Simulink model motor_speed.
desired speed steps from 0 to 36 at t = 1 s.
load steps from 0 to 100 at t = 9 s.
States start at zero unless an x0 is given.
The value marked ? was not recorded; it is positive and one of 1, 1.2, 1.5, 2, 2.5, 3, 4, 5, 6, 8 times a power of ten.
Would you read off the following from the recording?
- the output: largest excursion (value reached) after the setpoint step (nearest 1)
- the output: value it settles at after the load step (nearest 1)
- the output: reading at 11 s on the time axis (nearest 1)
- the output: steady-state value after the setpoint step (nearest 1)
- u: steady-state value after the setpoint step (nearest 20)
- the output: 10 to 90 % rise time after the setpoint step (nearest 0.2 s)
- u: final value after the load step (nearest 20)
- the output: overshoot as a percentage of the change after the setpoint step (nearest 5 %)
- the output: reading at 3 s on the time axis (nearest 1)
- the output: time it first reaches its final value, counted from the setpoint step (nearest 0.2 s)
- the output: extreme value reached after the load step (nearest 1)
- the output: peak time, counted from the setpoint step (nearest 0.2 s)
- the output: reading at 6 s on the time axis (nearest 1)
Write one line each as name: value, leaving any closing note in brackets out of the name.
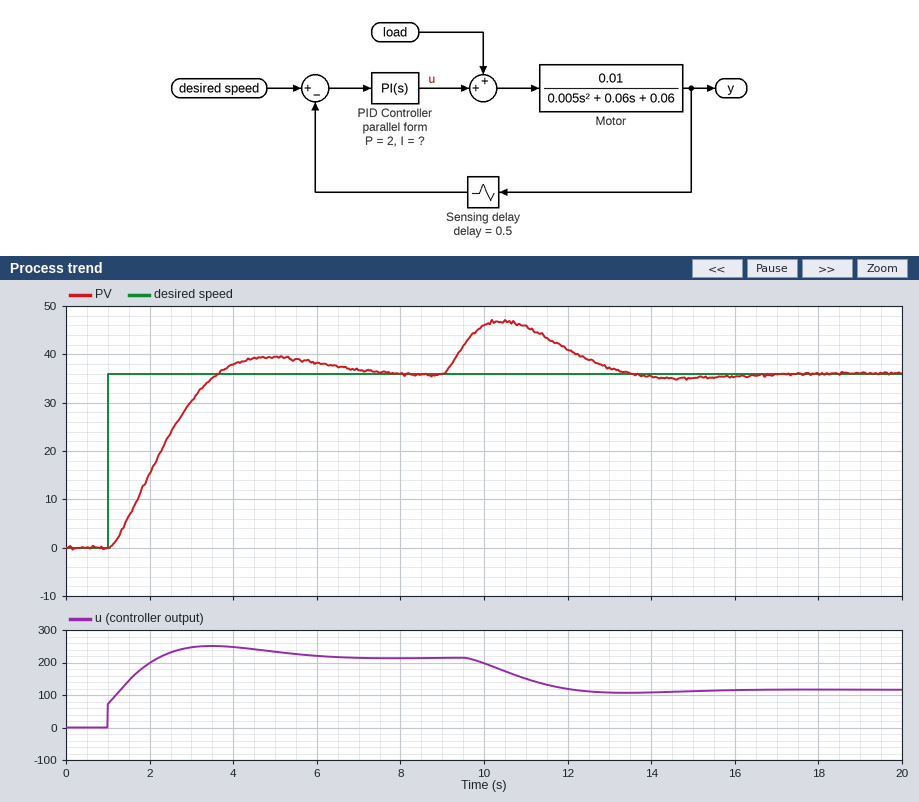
the output: largest excursion (value reached) after the setpoint step: 39
the output: value it settles at after the load step: 36
the output: reading at 11 s on the time axis: 46
the output: steady-state value after the setpoint step: 36
u: steady-state value after the setpoint step: 220
the output: 10 to 90 % rise time after the setpoint step: 1.8 s
u: final value after the load step: 120
the output: overshoot as a percentage of the change after the setpoint step: 10 %
the output: reading at 3 s on the time axis: 30
the output: time it first reaches its final value, counted from the setpoint step: 2.6 s
the output: extreme value reached after the load step: 47
the output: peak time, counted from the setpoint step: 3.8 s
the output: reading at 6 s on the time axis: 38
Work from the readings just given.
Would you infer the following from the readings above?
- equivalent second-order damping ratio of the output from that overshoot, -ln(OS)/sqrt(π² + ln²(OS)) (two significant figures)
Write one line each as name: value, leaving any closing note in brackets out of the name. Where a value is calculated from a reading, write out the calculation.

equivalent second-order damping ratio of the output from that overshoot, -ln(OS)/sqrt(π² + ln²(OS)): ln(0.1) = -2.303; 2.303 / sqrt(9.870 + 5.302) = 0.59
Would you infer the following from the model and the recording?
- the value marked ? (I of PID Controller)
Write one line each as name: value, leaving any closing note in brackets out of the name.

the value marked ?: 4
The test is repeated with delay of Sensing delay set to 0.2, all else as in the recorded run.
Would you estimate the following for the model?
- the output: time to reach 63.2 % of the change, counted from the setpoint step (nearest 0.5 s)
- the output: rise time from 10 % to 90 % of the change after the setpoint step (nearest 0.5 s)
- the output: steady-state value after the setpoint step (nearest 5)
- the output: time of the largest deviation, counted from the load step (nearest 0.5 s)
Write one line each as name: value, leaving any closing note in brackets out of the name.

the output: time to reach 63.2 % of the change, counted from the setpoint step: 1.5 s
the output: rise time from 10 % to 90 % of the change after the setpoint step: 2.5 s
the output: steady-state value after the setpoint step: 35
the output: time of the largest deviation, counted from the load step: 1.5 s
